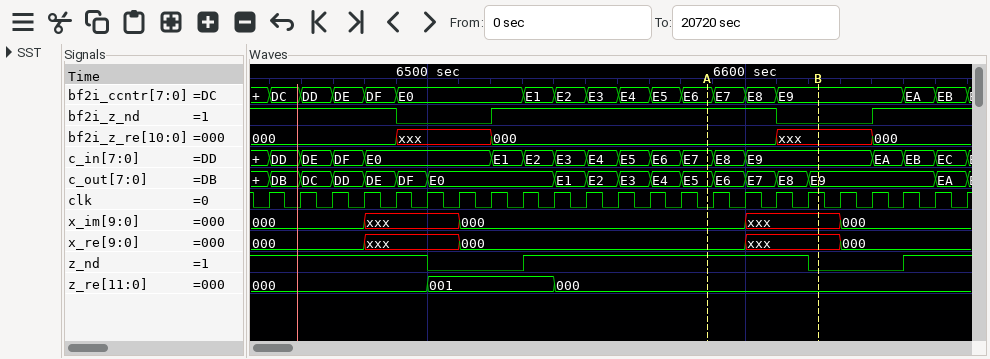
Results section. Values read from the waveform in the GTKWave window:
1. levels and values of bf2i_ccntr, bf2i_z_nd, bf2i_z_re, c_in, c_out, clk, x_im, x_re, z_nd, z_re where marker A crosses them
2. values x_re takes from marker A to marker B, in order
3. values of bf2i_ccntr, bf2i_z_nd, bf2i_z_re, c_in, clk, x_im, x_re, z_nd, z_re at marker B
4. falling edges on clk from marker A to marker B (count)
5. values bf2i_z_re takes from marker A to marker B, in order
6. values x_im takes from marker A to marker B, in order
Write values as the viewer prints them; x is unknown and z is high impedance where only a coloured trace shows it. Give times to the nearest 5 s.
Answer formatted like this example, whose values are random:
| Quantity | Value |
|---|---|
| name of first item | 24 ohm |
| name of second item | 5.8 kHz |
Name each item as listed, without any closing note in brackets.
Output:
| Quantity | Value |
|---|---|
| levels and values of bf2i_ccntr, bf2i_z_nd, bf2i_z_re, c_in, c_out, clk, x_im, x_re, z_nd, z_re where marker A crosses them | bf2i_ccntr=E6, bf2i_z_nd=1, bf2i_z_re=000, c_in=E7, c_out=E5, clk=0, x_im=000, x_re=000, z_nd=1, z_re=000 |
| values x_re takes from marker A to marker B, in order | 000, xxx |
| values of bf2i_ccntr, bf2i_z_nd, bf2i_z_re, c_in, clk, x_im, x_re, z_nd, z_re at marker B | bf2i_ccntr=E9, bf2i_z_nd=0, bf2i_z_re=xxx, c_in=E9, clk=1, x_im=xxx, x_re=xxx, z_nd=0, z_re=000 |
| falling edges on clk from marker A to marker B | 3 |
| values bf2i_z_re takes from marker A to marker B, in order | 000, xxx |
| values x_im takes from marker A to marker B, in order | 000, xxx |
